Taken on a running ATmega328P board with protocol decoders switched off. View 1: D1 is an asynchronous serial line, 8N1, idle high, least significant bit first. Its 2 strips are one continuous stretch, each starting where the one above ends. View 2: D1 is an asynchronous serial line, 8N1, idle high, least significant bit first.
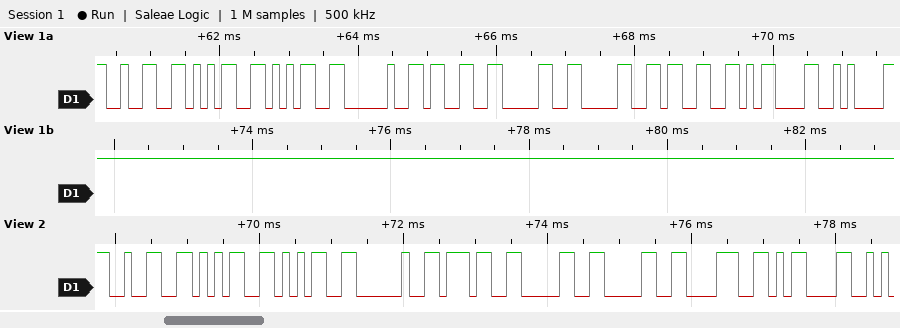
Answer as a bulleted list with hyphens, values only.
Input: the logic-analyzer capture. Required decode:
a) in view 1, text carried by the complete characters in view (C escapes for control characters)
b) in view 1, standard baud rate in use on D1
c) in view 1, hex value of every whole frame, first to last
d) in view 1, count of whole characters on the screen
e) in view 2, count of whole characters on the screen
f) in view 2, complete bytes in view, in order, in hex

- "255 3003\r\n"
- 9600 baud
- 0x32 0x35 0x35 0x20 0x33 0x30 0x30 0x33 0x0D 0x0A
- 10
- 9
- 32 35 35 20 37 30 30 38 0D
